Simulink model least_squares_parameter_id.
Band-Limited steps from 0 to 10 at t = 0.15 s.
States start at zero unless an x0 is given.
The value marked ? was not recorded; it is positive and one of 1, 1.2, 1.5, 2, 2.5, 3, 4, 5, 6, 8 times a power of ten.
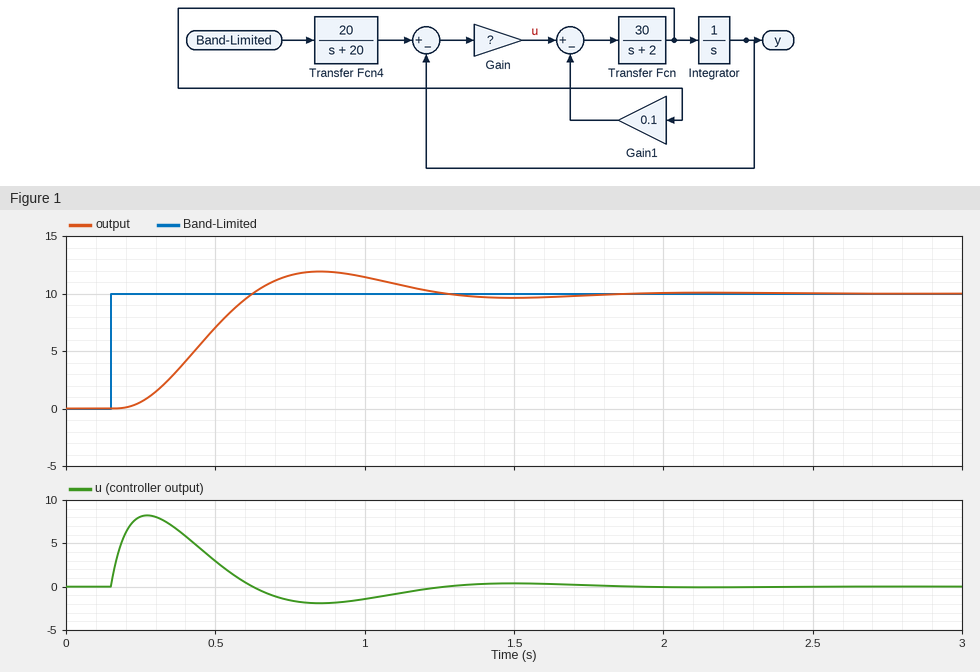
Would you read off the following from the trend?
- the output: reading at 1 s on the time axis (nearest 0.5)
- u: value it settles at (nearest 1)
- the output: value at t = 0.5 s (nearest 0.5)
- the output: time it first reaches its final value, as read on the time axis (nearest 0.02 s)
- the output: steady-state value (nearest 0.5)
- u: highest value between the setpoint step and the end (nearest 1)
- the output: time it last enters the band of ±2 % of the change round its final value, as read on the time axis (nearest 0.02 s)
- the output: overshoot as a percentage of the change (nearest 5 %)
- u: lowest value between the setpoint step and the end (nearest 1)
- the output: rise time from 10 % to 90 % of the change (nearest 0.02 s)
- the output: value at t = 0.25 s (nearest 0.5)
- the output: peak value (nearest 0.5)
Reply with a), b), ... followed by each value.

a) 11.5
b) 0
c) 7.0
d) 0.62 s
e) 10.0
f) 8
g) 1.72 s
h) 20 %
i) -2
j) 0.30 s
k) 0.5
l) 12.0
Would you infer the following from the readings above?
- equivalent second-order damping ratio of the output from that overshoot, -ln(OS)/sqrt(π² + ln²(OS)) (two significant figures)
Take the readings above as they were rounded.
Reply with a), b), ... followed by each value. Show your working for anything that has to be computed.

a) ln(0.2) = -1.609; 1.609 / sqrt(9.870 + 2.590) = 0.46
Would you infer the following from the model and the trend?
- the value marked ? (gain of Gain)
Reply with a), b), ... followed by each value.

a) 1
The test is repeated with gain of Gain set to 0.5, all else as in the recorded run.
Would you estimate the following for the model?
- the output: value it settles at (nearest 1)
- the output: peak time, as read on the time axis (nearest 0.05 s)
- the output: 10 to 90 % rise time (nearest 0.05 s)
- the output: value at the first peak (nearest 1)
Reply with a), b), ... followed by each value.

a) 10
b) 1.25 s
c) 0.50 s
d) 11
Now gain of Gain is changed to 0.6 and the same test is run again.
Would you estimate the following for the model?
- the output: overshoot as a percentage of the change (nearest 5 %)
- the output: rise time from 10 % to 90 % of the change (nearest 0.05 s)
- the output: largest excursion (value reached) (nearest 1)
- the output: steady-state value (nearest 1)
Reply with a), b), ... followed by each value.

a) 10 %
b) 0.45 s
c) 11
d) 10
